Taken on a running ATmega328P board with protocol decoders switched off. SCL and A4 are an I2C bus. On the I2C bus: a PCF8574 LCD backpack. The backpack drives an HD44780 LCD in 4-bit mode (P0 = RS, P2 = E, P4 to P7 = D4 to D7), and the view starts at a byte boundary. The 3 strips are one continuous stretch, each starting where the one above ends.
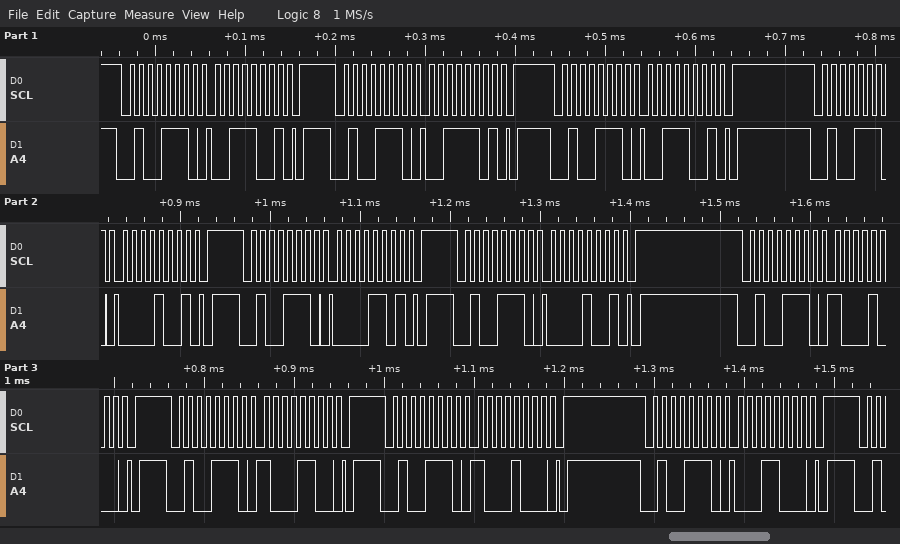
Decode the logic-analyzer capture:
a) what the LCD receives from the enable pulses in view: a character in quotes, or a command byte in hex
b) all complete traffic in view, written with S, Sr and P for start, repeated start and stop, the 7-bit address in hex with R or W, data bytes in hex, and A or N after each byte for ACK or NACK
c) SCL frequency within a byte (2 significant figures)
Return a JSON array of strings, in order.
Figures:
["'0'", "S 27W A 39 A P S 27W A 3D A P S 27W A 39 A P S 27W A 09 A P S 27W A 0D A P S 27W A 09 A P S 27W A 88 A P S 27W A 8C A P S 27W A 88 A P S 27W A 18 A P", "100 kHz"]
